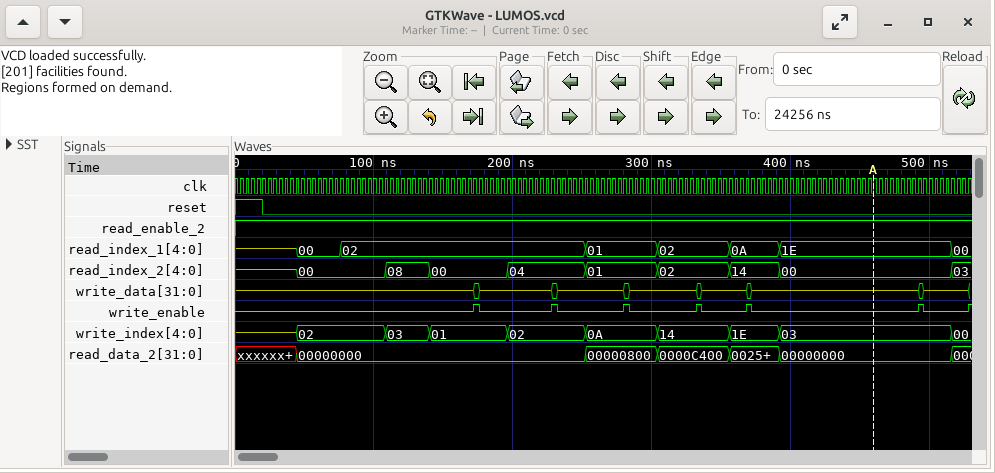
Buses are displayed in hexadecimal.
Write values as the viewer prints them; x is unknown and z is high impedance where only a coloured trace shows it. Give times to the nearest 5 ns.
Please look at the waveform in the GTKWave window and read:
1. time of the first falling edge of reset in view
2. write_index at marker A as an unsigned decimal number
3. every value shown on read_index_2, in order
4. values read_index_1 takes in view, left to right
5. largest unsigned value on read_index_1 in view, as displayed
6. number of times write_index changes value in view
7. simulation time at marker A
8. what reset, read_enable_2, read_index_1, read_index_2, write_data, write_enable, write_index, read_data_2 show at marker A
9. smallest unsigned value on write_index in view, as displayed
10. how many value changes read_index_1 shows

20 ns
3
z, 00, 08, 00, 04, 01, 02, 14, 00, 03
z, 00, 02, 01, 02, 0A, 1E, 00
1E
9
460 ns
reset=0, read_enable_2=1, read_index_1=1E, read_index_2=00, write_data=z, write_enable=z, write_index=03, read_data_2=00000000
00
7
